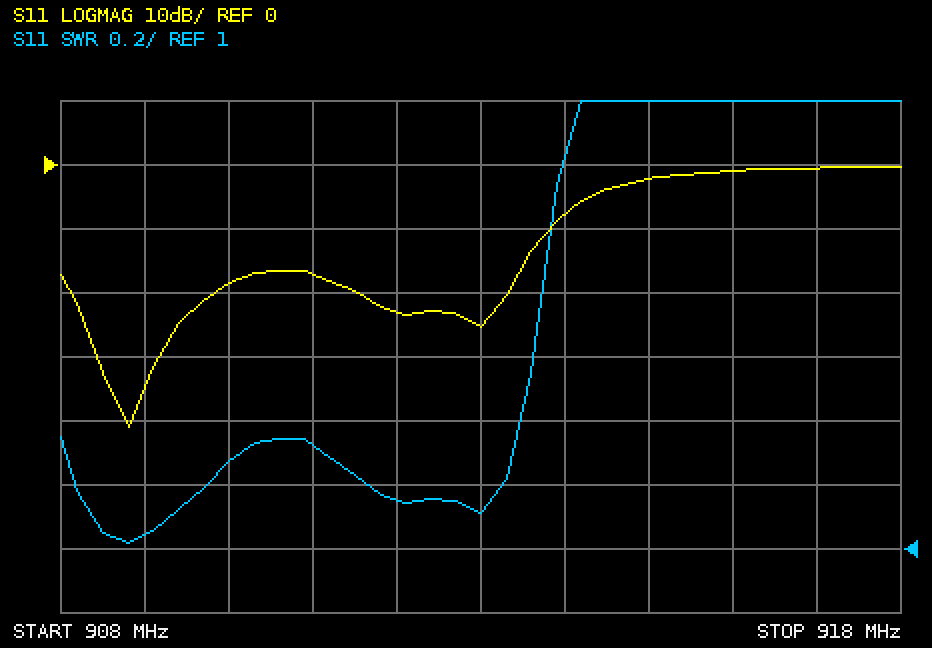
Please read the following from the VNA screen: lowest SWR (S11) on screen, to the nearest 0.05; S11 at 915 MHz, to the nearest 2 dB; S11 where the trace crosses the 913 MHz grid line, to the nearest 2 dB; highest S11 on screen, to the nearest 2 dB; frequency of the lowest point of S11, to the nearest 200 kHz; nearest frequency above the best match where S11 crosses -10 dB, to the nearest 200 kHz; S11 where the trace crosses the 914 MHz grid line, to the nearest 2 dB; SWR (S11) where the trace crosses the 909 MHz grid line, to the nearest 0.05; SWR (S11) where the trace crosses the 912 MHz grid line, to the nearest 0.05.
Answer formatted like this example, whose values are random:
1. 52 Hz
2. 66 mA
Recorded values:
1. 1.00
2. -2 dB
3. -26 dB
4. 0 dB
5. 908.8 MHz
6. 913.8 MHz
7. -8 dB
8. 1.05
9. 1.15
